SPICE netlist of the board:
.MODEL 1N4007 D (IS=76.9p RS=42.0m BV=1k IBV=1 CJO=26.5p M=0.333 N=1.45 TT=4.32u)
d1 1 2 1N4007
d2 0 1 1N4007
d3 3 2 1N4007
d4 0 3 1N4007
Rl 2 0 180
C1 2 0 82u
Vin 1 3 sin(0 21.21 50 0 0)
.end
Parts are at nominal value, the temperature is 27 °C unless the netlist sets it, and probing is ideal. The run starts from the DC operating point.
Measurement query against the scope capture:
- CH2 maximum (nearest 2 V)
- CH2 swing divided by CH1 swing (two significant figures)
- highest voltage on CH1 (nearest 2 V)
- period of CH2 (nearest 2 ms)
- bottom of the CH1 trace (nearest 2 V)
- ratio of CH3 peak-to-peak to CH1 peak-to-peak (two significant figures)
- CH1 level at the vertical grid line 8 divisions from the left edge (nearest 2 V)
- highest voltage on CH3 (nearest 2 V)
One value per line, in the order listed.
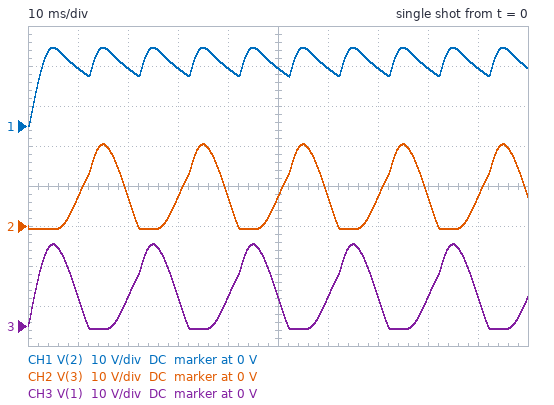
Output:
20 V
1.1
20 V
20 ms
0 V
1.1
14 V
20 V
